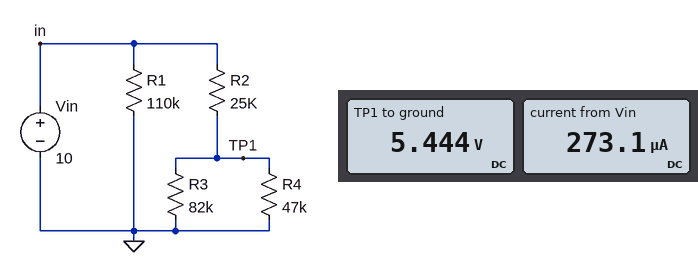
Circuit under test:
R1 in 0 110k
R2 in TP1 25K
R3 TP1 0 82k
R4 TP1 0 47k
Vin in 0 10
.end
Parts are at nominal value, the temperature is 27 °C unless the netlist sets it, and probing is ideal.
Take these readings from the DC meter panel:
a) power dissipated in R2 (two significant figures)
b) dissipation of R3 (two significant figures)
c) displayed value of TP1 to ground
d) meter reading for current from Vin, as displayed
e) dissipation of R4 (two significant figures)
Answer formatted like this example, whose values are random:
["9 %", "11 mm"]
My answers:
["830 µW", "360 µW", "5.444 V", "273.1 µA", "630 µW"]
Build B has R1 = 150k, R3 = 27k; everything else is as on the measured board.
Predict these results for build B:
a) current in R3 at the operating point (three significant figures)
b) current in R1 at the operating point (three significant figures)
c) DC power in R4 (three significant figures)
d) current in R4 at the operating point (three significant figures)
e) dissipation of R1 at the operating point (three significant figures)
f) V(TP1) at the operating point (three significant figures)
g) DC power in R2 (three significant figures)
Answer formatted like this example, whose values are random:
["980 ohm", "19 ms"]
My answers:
["151 µA", "66.7 µA", "352 µW", "86.6 µA", "667 µW", "4.07 V", "1.41 mW"]
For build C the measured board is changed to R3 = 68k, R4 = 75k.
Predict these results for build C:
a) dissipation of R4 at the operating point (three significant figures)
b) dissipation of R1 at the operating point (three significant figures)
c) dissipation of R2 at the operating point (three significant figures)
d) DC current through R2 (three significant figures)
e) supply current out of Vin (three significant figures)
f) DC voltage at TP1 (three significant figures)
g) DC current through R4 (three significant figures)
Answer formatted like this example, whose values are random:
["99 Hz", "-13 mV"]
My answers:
["461 µW", "909 µW", "679 µW", "165 µA", "256 µA", "5.88 V", "78.4 µA"]
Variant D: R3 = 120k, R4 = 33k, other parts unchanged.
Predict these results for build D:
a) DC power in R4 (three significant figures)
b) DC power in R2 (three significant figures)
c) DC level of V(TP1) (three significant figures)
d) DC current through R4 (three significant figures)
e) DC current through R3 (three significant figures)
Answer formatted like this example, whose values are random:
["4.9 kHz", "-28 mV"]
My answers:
["784 µW", "966 µW", "5.09 V", "154 µA", "42.4 µA"]
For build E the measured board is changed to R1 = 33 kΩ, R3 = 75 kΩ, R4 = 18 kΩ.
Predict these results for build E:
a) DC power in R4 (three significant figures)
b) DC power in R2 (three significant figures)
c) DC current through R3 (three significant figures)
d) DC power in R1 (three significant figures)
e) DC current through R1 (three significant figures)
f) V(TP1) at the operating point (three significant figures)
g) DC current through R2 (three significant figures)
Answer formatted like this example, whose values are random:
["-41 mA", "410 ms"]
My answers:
["750 µW", "1.60 mW", "49.0 µA", "3.03 mW", "303 µA", "3.67 V", "253 µA"]
